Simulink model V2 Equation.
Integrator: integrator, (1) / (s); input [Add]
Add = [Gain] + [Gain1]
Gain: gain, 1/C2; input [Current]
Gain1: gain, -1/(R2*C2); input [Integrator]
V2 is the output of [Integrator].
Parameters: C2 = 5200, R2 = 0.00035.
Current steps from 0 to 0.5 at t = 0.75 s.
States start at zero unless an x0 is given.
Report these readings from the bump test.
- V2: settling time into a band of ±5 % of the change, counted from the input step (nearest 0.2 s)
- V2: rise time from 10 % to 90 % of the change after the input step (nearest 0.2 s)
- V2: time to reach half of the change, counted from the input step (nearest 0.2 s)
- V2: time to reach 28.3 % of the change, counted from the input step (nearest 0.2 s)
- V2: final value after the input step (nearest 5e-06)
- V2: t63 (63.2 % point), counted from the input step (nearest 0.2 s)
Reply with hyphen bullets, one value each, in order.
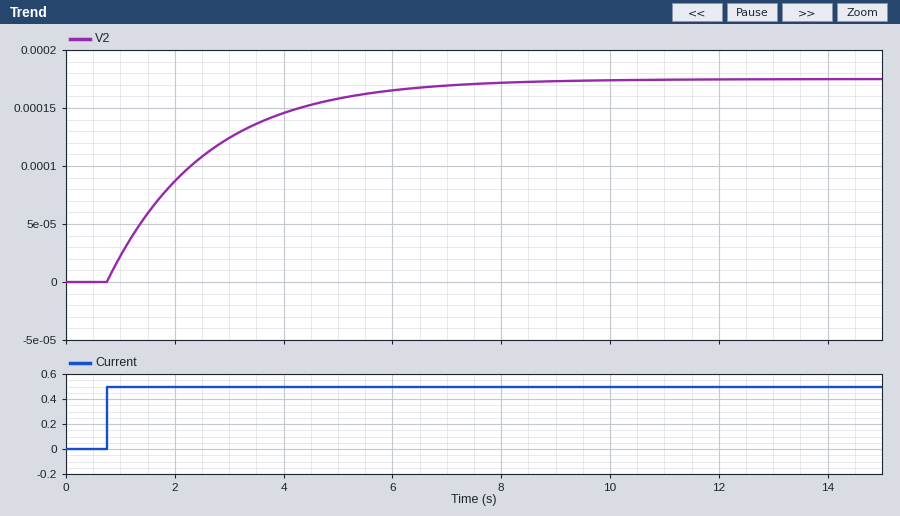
- 5.4 s
- 4.0 s
- 1.2 s
- 0.6 s
- 0.000175
- 1.8 s
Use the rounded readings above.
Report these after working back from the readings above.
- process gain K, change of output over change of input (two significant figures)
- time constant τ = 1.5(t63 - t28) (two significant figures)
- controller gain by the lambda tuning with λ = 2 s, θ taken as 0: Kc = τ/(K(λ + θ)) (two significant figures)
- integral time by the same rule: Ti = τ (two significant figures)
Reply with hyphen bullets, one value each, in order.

- 0.00035
- 1.8 s
- 2600
- 1.8 s
